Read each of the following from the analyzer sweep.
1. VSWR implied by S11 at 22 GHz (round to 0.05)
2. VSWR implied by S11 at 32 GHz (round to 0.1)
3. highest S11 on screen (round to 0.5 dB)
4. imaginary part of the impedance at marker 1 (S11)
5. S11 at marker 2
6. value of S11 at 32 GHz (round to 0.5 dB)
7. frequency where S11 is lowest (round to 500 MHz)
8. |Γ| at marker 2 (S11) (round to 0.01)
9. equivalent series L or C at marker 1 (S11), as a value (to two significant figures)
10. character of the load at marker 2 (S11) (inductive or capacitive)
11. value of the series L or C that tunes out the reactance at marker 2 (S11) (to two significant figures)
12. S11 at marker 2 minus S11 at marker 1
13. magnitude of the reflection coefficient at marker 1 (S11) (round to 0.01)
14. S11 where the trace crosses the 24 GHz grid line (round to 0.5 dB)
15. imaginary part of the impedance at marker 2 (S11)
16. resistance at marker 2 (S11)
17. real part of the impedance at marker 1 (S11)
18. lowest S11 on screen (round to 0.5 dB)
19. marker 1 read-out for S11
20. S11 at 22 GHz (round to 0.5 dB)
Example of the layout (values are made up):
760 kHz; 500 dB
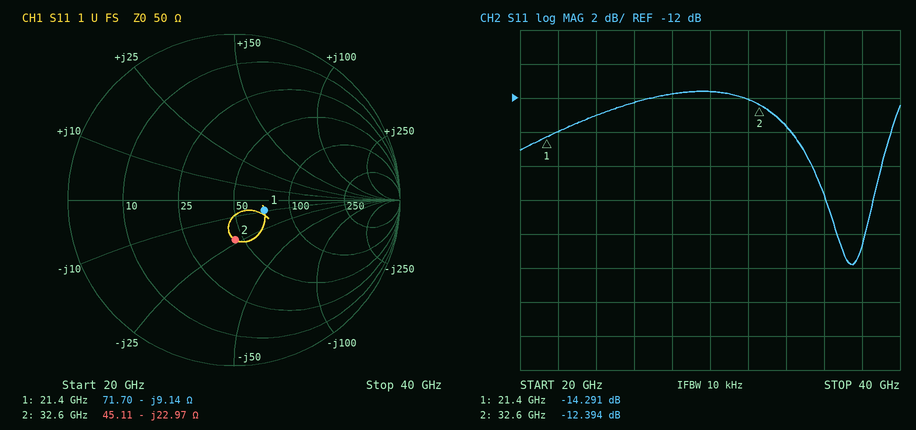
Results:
1.50; 1.7; -11.5 dB; -9.14 Ω; -12.394 dB; -12.0 dB; 37.5 GHz; 0.24; 810 fF; capacitive; 110 pH; 1.897 dB; 0.19; -13.0 dB; -22.97 Ω; 45.11 Ω; 71.70 Ω; -22.0 dB; -14.291 dB; -14.0 dB
